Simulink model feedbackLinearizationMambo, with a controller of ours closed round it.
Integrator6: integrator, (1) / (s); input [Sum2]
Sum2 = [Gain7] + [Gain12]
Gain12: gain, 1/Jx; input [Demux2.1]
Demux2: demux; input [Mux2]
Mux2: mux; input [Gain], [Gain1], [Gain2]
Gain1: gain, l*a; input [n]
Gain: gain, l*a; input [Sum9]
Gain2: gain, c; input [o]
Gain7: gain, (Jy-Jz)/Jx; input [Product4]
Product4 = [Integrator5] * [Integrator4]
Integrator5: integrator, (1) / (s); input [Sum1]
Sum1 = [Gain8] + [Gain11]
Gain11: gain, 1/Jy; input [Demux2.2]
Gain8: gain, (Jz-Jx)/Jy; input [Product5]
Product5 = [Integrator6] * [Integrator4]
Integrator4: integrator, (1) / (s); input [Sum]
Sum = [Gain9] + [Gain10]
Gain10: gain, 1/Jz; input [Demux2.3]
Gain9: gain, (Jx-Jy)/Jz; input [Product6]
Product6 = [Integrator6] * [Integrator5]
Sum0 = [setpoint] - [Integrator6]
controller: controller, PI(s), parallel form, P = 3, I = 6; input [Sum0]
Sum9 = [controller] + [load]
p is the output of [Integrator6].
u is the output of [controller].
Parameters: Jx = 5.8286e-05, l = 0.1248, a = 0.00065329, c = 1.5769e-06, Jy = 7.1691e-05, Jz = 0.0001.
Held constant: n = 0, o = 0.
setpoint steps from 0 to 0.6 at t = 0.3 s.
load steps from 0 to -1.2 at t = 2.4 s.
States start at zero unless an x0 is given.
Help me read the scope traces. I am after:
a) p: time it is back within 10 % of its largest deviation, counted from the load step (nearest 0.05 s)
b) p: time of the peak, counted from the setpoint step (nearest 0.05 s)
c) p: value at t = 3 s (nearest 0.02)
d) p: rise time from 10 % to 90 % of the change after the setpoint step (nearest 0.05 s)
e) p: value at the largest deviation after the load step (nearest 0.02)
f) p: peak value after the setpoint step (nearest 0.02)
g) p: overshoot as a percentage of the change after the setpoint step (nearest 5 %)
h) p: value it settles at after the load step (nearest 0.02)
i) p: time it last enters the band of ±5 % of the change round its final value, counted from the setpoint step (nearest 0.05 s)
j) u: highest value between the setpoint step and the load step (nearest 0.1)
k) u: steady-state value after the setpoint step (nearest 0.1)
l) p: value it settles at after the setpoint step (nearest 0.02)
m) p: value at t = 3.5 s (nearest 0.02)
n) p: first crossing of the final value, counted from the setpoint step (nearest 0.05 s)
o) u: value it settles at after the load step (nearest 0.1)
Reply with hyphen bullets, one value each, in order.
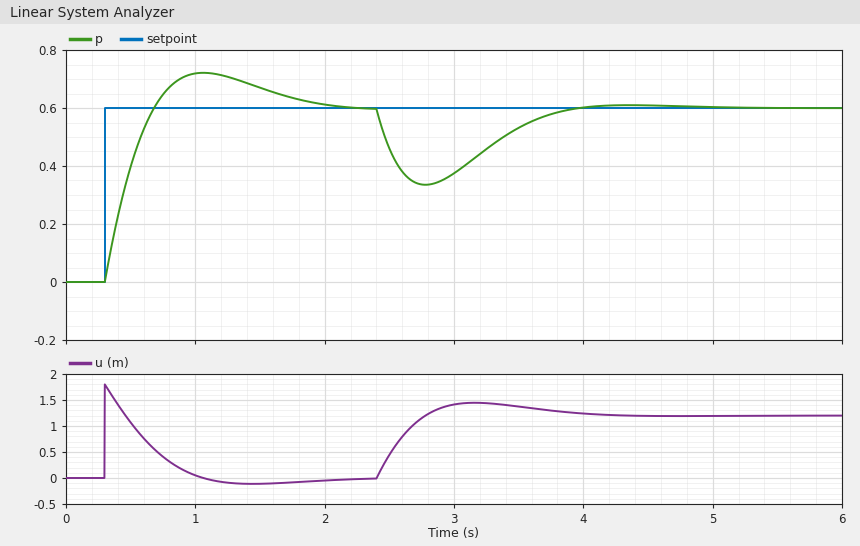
- 1.30 s
- 0.75 s
- 0.38
- 0.30 s
- 0.34
- 0.72
- 20 %
- 0.60
- 1.50 s
- 1.8
- 0.0
- 0.60
- 0.54
- 0.40 s
- 1.2
